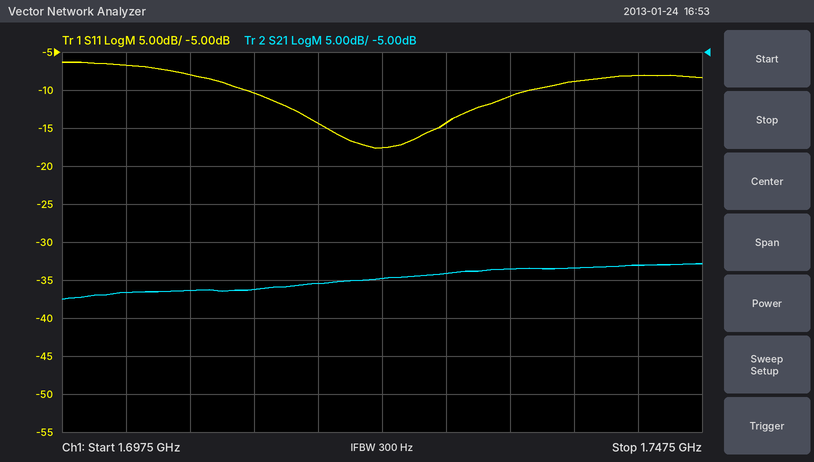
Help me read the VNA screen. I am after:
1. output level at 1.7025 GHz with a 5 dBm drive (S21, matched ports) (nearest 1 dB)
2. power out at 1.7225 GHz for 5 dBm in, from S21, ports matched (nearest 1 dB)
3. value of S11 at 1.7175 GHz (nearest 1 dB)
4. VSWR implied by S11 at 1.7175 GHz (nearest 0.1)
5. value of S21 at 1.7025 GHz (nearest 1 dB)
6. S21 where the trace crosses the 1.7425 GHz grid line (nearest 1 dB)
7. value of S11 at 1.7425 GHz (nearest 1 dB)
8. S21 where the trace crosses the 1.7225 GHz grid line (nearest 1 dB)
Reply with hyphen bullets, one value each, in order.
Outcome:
- -32 dBm
- -30 dBm
- -14 dB
- 1.5
- -37 dB
- -33 dB
- -8 dB
- -35 dB
